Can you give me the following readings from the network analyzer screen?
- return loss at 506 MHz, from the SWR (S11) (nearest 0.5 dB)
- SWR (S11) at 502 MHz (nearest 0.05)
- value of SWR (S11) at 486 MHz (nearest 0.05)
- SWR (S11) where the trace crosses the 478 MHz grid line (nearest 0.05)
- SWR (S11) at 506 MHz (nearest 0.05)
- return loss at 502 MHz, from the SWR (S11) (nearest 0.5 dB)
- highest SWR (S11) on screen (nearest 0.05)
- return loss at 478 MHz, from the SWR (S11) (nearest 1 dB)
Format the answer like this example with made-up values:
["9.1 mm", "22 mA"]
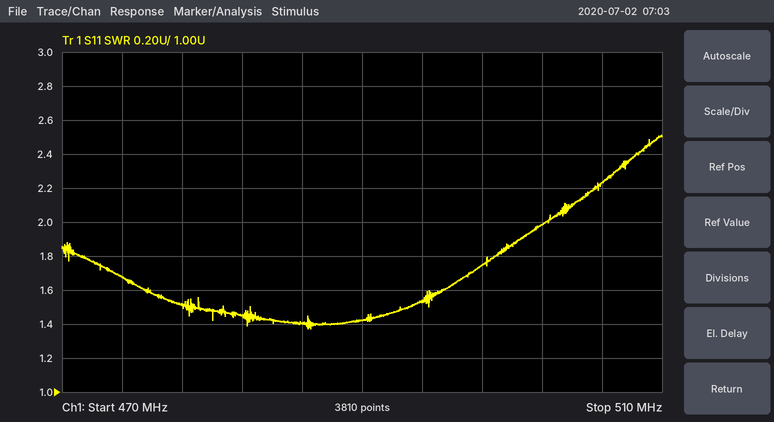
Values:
["8.5 dB", "2.00", "1.40", "1.50", "2.25", "9.5 dB", "2.50", "14 dB"]
